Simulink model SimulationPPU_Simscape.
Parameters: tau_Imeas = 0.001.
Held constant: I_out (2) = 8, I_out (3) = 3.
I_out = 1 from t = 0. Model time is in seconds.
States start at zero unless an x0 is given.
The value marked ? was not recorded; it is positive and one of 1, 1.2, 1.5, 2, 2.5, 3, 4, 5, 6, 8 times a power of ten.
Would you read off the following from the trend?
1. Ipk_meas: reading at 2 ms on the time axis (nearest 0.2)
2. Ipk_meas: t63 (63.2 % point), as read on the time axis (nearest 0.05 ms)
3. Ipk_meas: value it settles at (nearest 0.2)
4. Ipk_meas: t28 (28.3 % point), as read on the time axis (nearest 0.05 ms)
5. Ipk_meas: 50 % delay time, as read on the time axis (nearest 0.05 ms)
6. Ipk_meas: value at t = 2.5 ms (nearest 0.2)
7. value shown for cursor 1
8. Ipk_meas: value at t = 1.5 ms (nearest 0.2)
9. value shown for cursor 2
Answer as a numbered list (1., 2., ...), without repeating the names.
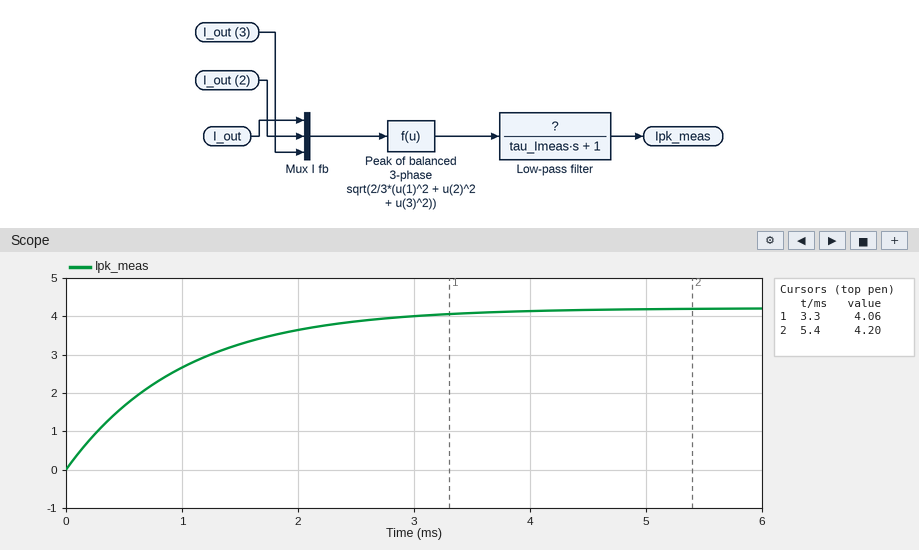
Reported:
1. 3.6
2. 1.00 ms
3. 4.2
4. 0.35 ms
5. 0.70 ms
6. 3.8
7. 4.06
8. 3.2
9. 4.20
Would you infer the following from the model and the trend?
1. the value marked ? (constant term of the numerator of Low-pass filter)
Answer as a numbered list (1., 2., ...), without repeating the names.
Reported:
1. 0.6
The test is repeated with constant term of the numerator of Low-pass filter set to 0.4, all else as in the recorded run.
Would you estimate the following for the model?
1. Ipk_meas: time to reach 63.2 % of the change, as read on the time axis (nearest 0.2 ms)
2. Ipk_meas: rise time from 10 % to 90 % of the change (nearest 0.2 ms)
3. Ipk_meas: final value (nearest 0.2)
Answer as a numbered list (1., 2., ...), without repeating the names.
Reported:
1. 1.0 ms
2. 2.2 ms
3. 2.8
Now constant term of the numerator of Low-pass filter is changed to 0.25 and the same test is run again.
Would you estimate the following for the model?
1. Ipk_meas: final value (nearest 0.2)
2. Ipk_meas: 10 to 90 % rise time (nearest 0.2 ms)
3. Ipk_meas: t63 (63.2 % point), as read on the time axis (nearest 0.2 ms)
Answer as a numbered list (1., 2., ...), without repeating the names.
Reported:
1. 1.8
2. 2.2 ms
3. 1.0 ms
